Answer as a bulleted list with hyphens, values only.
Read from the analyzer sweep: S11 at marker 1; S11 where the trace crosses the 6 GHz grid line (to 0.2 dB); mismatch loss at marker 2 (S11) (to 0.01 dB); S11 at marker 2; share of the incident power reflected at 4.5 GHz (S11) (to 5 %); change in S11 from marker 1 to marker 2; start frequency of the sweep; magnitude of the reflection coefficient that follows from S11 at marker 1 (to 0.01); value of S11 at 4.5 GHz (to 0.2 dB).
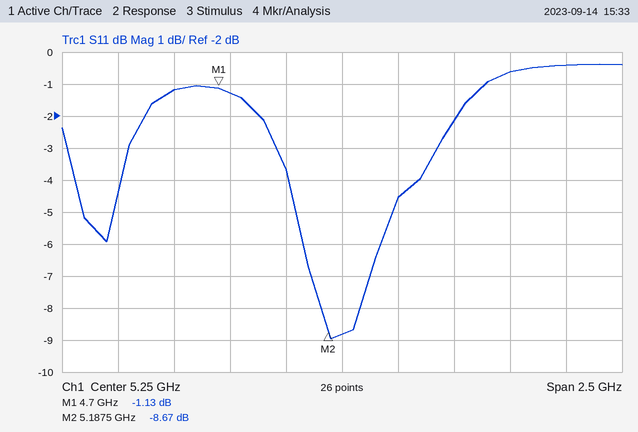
- -1.13 dB
- -0.6 dB
- 0.63 dB
- -8.67 dB
- 75 %
- -7.54 dB
- 4 GHz
- 0.88
- -1.2 dB
